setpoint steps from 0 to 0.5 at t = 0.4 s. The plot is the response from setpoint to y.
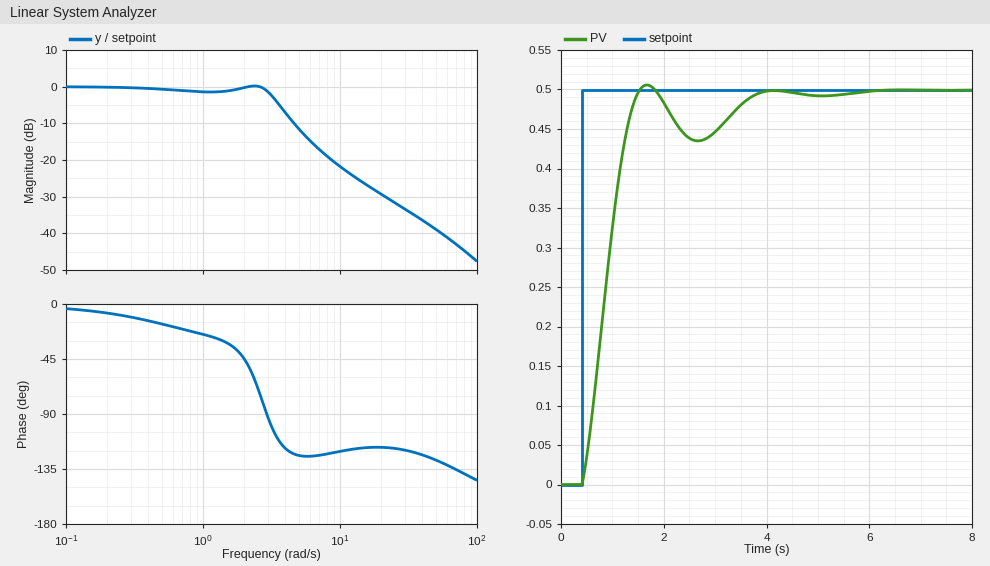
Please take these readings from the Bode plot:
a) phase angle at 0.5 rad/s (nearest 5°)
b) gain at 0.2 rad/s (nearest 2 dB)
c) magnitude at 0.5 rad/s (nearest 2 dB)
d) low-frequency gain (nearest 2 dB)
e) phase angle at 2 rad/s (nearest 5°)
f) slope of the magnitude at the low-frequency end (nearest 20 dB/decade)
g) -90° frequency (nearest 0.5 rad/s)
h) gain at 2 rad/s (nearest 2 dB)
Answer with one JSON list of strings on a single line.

["-15°", "0 dB", "0 dB", "0 dB", "-45°", "0 dB/decade", "3.0 rad/s", "0 dB"]
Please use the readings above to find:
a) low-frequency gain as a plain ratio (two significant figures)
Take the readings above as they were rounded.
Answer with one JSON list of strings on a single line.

["1.0"]
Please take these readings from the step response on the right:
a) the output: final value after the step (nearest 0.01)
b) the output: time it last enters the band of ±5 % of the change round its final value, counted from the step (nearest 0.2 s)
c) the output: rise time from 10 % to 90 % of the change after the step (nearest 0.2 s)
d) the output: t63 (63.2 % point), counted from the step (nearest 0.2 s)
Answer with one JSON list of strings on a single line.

["0.50", "3.0 s", "0.8 s", "0.6 s"]
